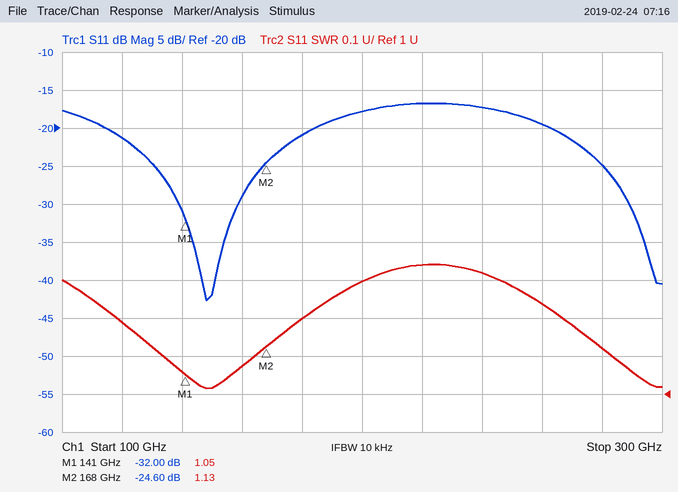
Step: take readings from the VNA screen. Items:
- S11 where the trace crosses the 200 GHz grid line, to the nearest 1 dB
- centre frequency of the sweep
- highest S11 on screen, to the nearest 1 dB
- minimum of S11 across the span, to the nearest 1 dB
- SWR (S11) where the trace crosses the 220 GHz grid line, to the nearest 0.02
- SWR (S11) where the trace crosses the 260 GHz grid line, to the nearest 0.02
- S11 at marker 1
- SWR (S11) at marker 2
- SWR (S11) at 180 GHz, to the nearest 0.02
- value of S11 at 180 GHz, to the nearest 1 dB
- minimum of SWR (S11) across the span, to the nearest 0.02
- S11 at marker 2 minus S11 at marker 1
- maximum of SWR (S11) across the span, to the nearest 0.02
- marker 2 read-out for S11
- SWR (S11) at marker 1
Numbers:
-18 dB
200 GHz
-17 dB
-43 dB
1.34
1.24
-32.00 dB
1.13
1.20
-21 dB
1.02
7.40 dB
1.34
-24.60 dB
1.05
